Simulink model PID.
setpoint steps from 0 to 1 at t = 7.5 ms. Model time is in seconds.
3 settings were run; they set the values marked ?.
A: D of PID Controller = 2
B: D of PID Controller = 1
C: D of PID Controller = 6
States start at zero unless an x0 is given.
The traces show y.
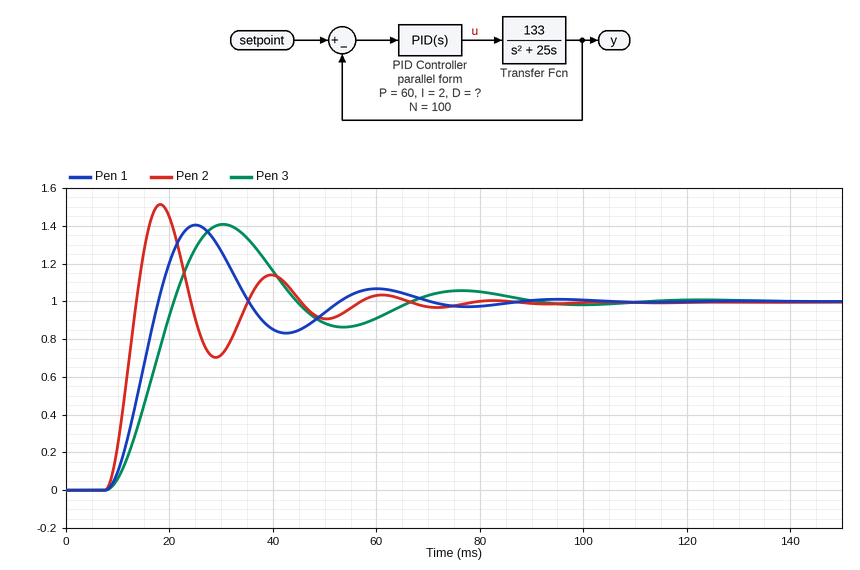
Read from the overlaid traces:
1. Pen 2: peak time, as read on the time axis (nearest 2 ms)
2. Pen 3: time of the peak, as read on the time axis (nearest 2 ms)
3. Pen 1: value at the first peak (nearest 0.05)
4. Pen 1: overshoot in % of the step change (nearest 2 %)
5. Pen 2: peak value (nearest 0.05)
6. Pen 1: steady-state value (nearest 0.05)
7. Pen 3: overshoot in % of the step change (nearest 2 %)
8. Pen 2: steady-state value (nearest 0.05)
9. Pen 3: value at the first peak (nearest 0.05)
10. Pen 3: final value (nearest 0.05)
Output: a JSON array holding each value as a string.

["18 ms", "30 ms", "1.40", "40 %", "1.50", "1.00", "40 %", "1.00", "1.40", "1.00"]
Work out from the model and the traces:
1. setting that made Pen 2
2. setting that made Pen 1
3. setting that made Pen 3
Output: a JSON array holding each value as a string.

["C", "A", "B"]
